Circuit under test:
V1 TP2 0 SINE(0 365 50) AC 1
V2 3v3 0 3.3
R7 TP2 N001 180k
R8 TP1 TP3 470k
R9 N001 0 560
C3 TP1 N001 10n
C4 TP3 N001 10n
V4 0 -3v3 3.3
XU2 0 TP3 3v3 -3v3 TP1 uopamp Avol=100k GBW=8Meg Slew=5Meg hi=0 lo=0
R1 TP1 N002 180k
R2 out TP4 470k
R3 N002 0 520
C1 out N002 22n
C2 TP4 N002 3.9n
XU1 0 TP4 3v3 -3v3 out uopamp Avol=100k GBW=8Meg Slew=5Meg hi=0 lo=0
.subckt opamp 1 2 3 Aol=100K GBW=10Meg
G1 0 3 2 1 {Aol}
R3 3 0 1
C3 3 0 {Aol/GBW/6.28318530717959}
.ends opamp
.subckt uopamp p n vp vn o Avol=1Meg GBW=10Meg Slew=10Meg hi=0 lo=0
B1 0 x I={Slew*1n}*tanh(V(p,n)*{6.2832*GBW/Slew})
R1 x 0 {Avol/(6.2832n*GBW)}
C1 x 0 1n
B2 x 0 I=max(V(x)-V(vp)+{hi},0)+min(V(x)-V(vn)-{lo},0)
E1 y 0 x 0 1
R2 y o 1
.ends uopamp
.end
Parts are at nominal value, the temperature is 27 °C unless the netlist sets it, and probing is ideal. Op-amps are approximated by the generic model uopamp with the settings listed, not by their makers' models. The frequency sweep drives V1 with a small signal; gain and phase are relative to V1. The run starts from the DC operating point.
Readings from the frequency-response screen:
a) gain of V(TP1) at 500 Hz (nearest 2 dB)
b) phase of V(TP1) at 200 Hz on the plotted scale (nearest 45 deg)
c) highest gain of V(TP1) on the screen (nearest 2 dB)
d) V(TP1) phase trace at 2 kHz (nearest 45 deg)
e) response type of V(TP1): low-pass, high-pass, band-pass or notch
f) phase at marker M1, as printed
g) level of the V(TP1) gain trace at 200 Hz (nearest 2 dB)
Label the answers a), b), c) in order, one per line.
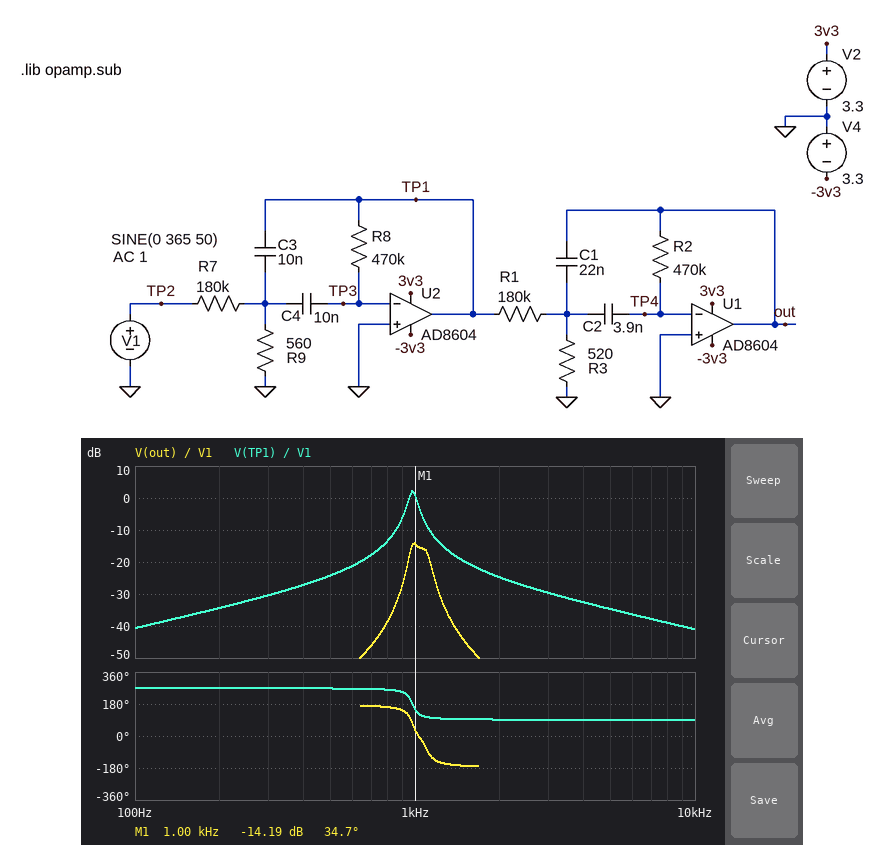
a) -24 dB
b) 270 deg
c) 2 dB
d) 90 deg
e) band-pass
f) 34.7 deg
g) -34 dB
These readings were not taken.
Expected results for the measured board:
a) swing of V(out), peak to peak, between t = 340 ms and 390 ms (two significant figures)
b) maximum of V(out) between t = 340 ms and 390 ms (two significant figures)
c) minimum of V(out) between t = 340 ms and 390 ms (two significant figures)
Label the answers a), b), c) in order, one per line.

a) 5.6 mV
b) 2.8 mV
c) -2.8 mV
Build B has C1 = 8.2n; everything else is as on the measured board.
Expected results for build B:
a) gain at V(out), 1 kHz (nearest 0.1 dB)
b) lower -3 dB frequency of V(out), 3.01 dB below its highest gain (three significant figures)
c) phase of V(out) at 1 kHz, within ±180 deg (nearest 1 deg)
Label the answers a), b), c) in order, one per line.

a) -25.3 dB
b) 951 Hz
c) 57 deg
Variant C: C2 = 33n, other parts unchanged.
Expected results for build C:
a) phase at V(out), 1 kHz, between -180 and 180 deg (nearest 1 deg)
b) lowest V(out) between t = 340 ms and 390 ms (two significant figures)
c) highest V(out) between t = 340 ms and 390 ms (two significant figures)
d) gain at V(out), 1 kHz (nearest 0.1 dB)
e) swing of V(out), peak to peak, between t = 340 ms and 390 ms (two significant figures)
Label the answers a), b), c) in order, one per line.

a) -118 deg
b) -24 mV
c) 24 mV
d) -25.5 dB
e) 48 mV
